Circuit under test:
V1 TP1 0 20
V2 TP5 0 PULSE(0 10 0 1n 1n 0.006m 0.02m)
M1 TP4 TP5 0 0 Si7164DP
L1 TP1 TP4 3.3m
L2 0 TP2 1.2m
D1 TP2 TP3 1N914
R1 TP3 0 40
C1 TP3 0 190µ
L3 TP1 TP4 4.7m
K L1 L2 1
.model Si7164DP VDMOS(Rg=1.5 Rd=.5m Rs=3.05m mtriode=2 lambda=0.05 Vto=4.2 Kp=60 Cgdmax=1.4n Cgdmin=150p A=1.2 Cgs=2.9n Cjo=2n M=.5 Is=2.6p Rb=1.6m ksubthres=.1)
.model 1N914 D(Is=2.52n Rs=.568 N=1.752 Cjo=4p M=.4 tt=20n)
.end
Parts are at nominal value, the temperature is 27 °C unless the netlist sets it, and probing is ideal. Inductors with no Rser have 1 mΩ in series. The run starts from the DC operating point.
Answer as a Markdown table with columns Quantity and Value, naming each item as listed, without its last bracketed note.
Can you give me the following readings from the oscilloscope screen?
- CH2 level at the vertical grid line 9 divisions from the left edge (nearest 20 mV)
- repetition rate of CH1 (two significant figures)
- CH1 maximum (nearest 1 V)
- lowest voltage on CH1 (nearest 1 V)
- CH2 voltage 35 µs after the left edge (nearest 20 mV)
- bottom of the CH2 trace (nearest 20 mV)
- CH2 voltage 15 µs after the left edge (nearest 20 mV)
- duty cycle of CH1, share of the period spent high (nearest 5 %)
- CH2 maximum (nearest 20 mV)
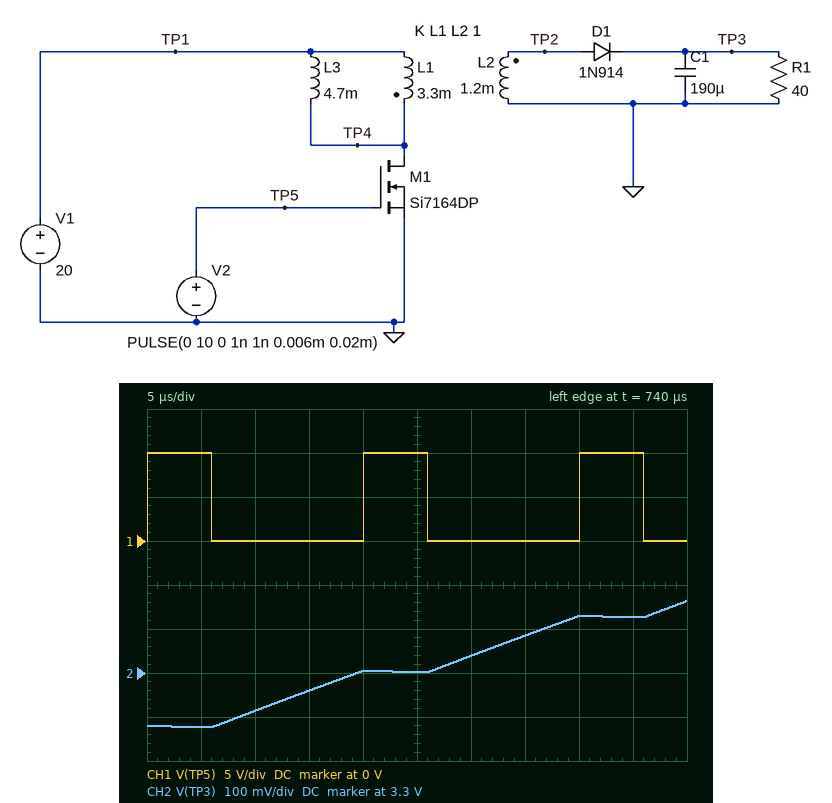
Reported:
| Quantity | Value |
|---|---|
| CH2 level at the vertical grid line 9 divisions from the left edge | 3.42 V |
| repetition rate of CH1 | 50 kHz |
| CH1 maximum | 10 V |
| lowest voltage on CH1 | 0 V |
| CH2 voltage 35 µs after the left edge | 3.38 V |
| bottom of the CH2 trace | 3.18 V |
| CH2 voltage 15 µs after the left edge | 3.26 V |
| duty cycle of CH1, share of the period spent high | 30 % |
| CH2 maximum | 3.46 V |
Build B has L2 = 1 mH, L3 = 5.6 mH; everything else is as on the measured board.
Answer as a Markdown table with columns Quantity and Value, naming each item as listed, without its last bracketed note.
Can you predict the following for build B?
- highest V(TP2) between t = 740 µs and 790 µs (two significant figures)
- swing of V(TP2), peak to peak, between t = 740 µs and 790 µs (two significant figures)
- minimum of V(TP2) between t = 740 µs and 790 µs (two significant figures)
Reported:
| Quantity | Value |
|---|---|
| highest V(TP2) between t = 740 µs and 790 µs | 5.4 V |
| swing of V(TP2), peak to peak, between t = 740 µs and 790 µs | 16 V |
| minimum of V(TP2) between t = 740 µs and 790 µs | -11 V |
